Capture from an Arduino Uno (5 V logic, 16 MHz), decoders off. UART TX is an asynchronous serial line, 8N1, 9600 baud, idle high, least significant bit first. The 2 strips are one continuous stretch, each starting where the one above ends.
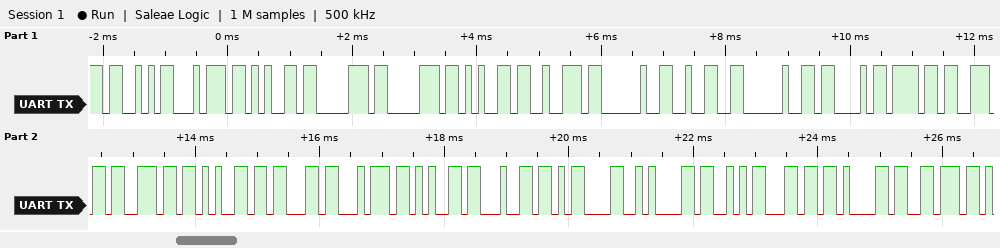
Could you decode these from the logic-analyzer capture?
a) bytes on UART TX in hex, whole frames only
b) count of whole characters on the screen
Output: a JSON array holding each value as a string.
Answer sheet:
["53 74 65 70 70 65 72 20 32 20 43 6F 6E 6E 65 63 74 65 64 0D 0A 53 6C 61 76", "25"]
